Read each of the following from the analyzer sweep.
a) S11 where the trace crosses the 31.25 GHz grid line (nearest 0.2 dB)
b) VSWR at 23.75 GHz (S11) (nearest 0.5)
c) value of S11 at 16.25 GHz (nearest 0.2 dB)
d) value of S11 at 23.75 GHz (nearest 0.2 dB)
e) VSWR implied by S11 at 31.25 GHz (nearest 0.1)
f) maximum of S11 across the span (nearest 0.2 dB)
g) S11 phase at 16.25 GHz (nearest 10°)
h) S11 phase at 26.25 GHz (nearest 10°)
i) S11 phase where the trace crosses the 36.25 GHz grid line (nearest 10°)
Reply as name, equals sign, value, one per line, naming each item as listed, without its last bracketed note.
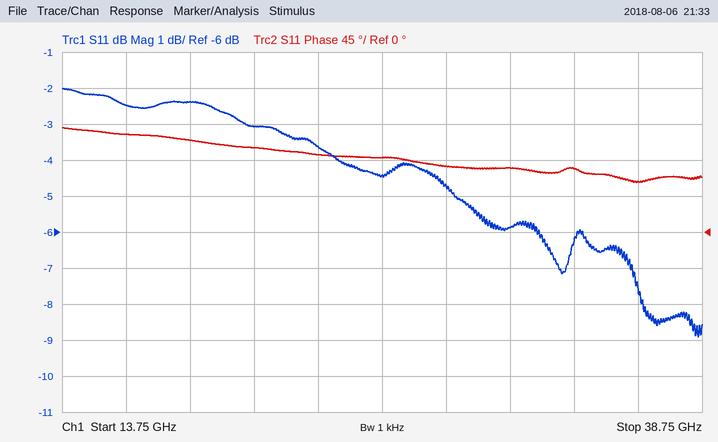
S11 where the trace crosses the 31.25 GHz grid line = -5.8 dB
VSWR at 23.75 GHz (S11) = 5.0
value of S11 at 16.25 GHz = -2.4 dB
value of S11 at 23.75 GHz = -3.6 dB
VSWR implied by S11 at 31.25 GHz = 3.1
maximum of S11 across the span = -2.0 dB
S11 phase at 16.25 GHz = 120°
S11 phase at 26.25 GHz = 90°
S11 phase where the trace crosses the 36.25 GHz grid line = 60°
